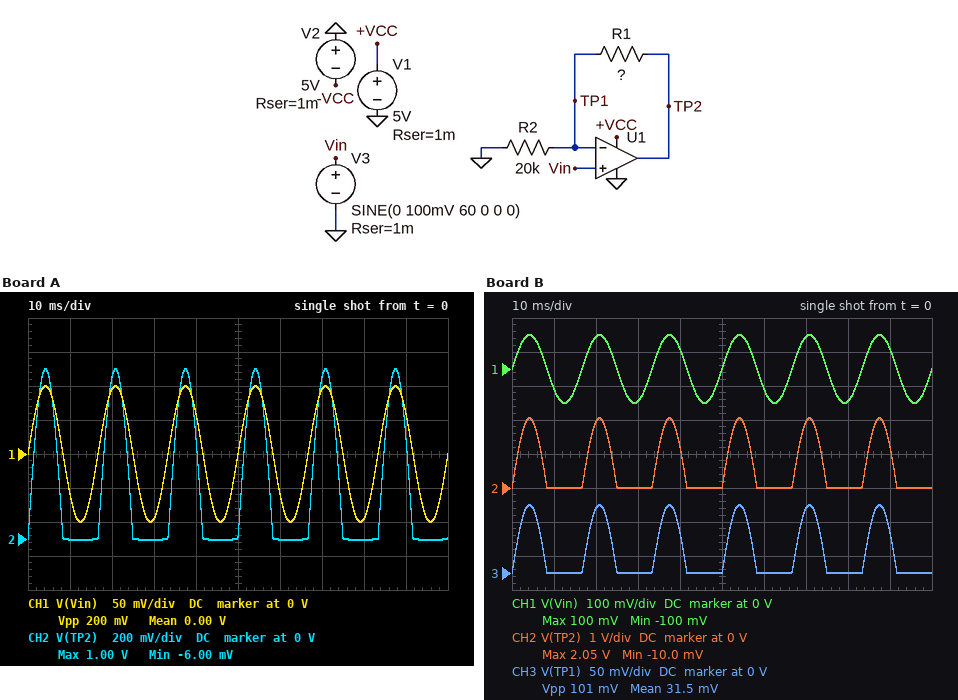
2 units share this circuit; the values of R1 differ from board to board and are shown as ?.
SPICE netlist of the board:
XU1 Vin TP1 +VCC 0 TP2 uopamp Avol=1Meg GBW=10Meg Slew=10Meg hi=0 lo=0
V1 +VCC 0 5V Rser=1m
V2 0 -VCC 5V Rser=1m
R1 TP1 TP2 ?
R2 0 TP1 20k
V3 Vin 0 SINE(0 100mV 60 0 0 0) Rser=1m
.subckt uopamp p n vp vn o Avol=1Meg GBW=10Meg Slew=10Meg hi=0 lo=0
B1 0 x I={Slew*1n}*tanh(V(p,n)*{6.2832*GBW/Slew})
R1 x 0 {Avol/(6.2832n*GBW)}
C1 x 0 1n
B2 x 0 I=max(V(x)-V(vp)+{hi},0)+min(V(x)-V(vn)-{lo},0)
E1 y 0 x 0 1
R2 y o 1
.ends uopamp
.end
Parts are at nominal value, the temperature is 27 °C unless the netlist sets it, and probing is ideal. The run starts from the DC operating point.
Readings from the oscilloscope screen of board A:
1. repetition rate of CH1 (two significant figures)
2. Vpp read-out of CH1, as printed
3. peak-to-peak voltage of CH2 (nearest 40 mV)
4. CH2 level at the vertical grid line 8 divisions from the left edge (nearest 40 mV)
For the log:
60 Hz
200 mV
1.00 V
0 V
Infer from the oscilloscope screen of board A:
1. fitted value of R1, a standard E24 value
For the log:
180 kΩ
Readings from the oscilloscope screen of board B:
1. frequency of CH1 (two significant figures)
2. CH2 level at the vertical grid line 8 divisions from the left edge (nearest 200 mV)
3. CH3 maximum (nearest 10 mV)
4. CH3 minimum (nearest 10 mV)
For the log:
60 Hz
0 V
100 mV
0 V
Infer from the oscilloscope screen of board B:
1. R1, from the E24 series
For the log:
390 kΩ
